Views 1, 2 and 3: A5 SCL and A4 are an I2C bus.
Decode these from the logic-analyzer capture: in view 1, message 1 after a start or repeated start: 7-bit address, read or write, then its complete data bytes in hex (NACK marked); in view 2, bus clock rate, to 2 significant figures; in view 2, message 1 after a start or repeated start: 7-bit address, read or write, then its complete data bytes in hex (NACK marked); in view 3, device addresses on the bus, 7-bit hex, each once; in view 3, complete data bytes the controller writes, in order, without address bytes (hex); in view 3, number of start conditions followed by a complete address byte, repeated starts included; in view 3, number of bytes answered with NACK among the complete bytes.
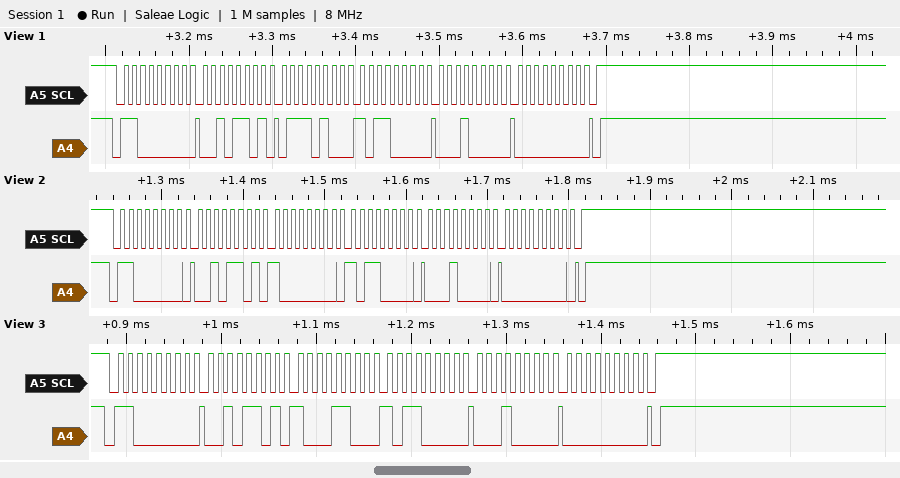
0x60 write: 2D 74 B0 10 00
100 kHz
0x60 write: 2D 80 B0 10 00
0x60
2D 8C B0 10 00
1
0
